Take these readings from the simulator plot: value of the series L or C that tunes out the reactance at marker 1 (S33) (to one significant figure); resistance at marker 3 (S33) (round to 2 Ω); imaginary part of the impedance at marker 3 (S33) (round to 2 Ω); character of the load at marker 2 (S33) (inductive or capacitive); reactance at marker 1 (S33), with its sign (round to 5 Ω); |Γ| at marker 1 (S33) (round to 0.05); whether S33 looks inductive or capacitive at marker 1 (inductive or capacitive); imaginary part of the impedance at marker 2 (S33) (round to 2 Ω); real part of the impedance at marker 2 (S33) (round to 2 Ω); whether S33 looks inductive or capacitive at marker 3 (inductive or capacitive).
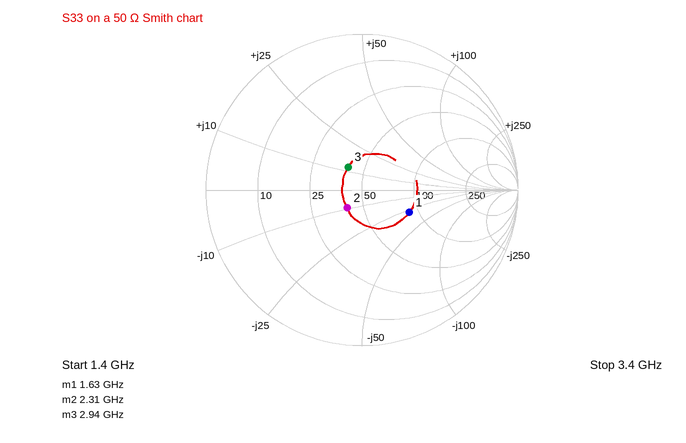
3 nH
40 Ω
+12 Ω
capacitive
-30 Ω
0.35
capacitive
-10 Ω
40 Ω
inductive
